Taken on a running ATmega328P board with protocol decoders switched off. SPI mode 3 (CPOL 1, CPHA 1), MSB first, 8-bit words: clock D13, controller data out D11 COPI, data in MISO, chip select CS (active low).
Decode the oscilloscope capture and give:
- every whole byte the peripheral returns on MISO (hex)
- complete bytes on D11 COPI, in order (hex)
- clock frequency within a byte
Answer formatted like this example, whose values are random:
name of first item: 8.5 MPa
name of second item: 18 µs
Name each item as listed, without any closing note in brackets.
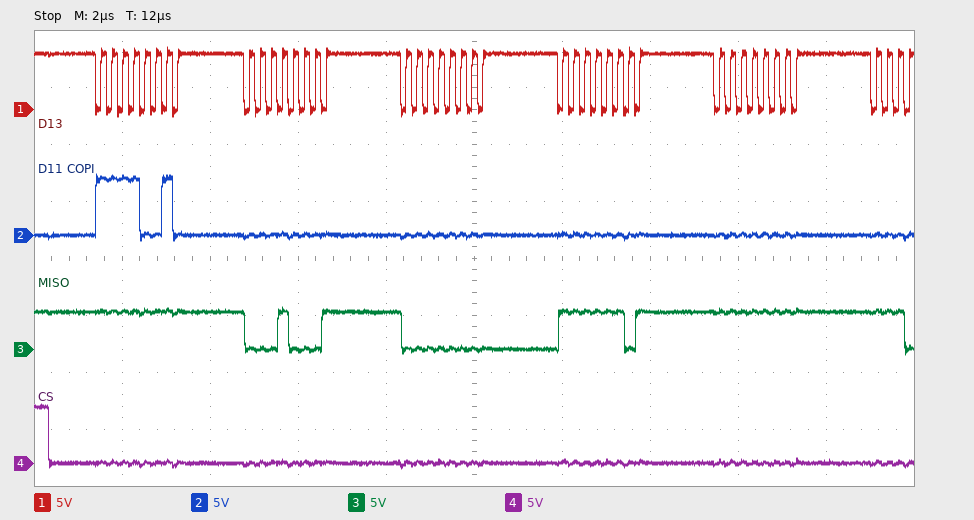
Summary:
every whole byte the peripheral returns on MISO: 0xFF 0x11 0x00 0xFD 0xFF
complete bytes on D11 COPI, in order: 0xF2 0x00 0x00 0x00 0x00
clock frequency within a byte: 4 MHz
